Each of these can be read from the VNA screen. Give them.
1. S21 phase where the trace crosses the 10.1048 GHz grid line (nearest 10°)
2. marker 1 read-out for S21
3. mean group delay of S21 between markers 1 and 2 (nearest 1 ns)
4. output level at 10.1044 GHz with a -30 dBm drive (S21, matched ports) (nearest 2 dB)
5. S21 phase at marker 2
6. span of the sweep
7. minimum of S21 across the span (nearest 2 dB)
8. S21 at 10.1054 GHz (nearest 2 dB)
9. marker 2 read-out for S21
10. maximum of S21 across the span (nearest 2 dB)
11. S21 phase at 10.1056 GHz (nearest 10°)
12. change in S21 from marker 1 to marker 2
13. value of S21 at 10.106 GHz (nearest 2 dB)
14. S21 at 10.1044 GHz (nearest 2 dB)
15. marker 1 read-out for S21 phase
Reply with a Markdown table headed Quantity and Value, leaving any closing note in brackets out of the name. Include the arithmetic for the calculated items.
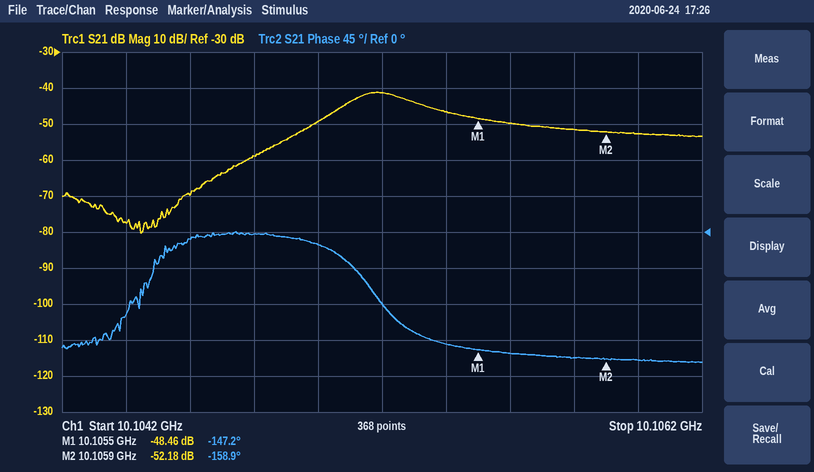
| Quantity | Value |
|---|---|
| S21 phase where the trace crosses the 10.1048 GHz grid line | 0° |
| marker 1 read-out for S21 | -48.46 dB |
| mean group delay of S21 between markers 1 and 2 | −(-158.9° − (-147.2°))/(360° × 400 kHz) ≈ 81 ns |
| output level at 10.1044 GHz with a -30 dBm drive (S21, matched ports) | -30 dBm + (-78 dB) = -108 dBm |
| S21 phase at marker 2 | -158.9° |
| span of the sweep | 2 MHz |
| minimum of S21 across the span | -80 dB |
| S21 at 10.1054 GHz | -46 dB |
| marker 2 read-out for S21 | -52.18 dB |
| maximum of S21 across the span | -42 dB |
| S21 phase at 10.1056 GHz | -150° |
| change in S21 from marker 1 to marker 2 | -52.18 − (-48.46) = -3.72 dB |
| value of S21 at 10.106 GHz | -52 dB |
| S21 at 10.1044 GHz | -78 dB |
| marker 1 read-out for S21 phase | -147.2° |
